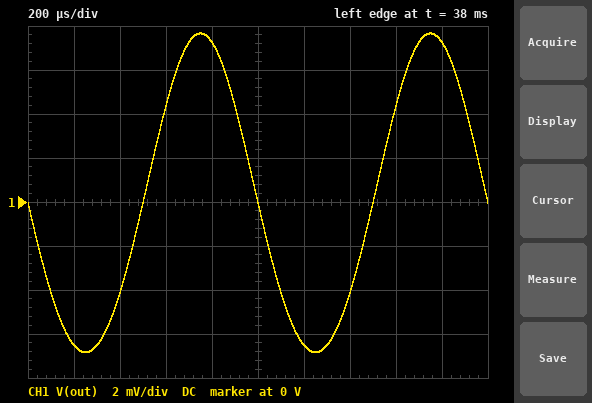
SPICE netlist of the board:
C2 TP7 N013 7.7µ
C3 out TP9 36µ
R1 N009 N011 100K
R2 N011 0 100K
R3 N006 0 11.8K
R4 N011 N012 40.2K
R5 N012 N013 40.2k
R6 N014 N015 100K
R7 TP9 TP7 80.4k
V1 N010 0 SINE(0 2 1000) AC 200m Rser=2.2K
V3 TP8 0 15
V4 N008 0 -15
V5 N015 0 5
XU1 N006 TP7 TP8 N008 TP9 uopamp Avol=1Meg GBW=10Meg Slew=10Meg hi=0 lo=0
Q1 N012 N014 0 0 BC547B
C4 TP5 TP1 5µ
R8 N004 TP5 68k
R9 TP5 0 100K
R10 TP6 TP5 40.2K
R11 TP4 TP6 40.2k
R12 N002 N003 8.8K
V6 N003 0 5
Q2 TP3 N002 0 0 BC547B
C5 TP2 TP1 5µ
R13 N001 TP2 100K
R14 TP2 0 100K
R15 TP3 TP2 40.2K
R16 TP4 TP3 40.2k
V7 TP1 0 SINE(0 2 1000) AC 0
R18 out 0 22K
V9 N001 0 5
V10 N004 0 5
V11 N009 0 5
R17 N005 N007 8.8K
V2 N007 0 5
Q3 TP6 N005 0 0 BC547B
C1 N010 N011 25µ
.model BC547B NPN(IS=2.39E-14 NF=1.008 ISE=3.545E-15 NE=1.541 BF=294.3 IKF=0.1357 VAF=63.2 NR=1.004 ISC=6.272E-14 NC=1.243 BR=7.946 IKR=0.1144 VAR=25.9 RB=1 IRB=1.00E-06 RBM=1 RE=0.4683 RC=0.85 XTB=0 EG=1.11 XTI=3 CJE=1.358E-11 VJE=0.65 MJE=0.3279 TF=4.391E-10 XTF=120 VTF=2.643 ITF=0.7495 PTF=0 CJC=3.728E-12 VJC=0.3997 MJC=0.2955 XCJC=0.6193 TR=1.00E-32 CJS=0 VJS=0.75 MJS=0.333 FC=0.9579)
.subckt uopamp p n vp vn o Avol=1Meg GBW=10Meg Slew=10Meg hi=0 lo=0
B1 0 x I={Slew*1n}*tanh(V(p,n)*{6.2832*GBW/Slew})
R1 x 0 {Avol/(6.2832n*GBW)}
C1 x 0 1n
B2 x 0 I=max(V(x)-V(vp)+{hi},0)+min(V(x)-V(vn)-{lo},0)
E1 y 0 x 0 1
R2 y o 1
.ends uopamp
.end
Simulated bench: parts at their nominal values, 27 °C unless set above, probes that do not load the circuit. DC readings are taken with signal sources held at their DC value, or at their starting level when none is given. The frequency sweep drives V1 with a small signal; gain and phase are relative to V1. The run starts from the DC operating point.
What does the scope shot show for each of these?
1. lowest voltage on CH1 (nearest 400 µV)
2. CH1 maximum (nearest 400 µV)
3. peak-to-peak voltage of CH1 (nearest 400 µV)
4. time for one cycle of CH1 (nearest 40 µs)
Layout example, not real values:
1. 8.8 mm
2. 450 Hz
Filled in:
1. -6.8 mV
2. 7.6 mV
3. 14.4 mV
4. 1.00 ms
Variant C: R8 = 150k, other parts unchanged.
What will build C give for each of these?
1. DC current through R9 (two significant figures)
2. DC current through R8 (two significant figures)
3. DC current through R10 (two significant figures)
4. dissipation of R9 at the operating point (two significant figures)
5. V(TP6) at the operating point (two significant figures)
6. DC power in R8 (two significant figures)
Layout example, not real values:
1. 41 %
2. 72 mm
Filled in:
1. 8.1 µA
2. 28 µA
3. 20 µA
4. 6.5 µW
5. 6.9 mV
6. 120 µW
